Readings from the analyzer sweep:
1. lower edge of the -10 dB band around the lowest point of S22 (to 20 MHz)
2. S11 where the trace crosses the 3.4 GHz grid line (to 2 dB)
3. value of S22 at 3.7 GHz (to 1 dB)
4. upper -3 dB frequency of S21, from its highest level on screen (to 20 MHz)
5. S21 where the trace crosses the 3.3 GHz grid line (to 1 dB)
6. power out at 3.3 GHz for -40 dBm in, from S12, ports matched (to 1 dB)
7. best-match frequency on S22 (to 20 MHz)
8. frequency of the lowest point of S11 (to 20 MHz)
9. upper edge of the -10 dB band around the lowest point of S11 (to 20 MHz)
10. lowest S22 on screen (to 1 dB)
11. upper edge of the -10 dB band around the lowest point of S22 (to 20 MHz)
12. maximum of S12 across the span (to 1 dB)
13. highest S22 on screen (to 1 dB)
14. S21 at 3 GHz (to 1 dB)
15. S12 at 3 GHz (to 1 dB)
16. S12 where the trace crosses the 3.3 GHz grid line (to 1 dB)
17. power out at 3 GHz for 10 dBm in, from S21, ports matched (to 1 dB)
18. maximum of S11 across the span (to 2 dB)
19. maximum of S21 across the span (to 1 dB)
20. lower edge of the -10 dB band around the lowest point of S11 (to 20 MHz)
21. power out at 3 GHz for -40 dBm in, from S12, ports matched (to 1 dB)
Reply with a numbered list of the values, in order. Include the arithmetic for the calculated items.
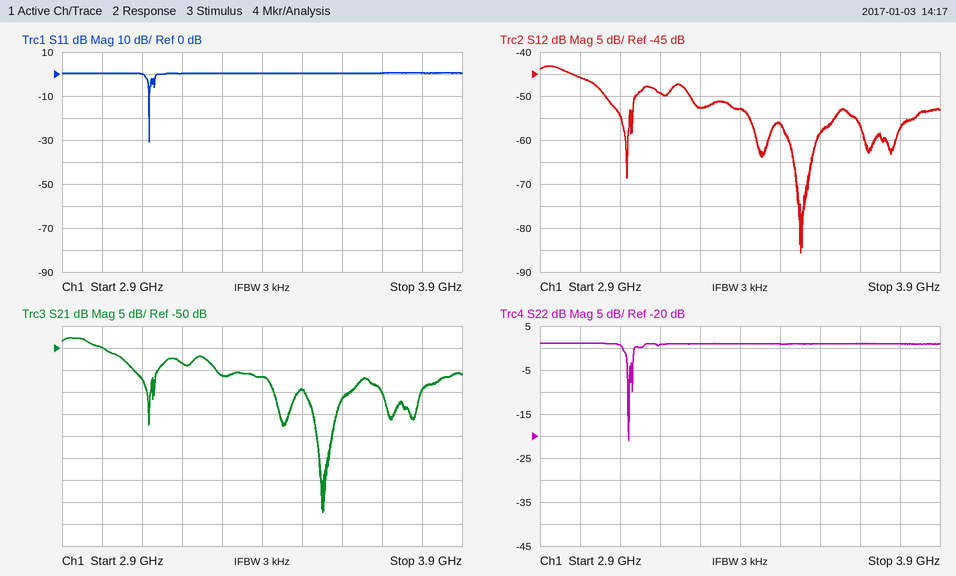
1. 3.12 GHz
2. 0 dB
3. 1 dB
4. 3.02 GHz
5. -56 dB
6. -40 dBm + (-53 dB) = -93 dBm
7. 3.12 GHz
8. 3.12 GHz
9. 3.12 GHz
10. -21 dB
11. 3.12 GHz
12. -43 dB
13. 1 dB
14. -50 dB
15. -46 dB
16. -53 dB
17. 10 dBm + (-50 dB) = -40 dBm
18. 0 dB
19. -48 dB
20. 3.12 GHz
21. -40 dBm + (-46 dB) = -86 dBm
